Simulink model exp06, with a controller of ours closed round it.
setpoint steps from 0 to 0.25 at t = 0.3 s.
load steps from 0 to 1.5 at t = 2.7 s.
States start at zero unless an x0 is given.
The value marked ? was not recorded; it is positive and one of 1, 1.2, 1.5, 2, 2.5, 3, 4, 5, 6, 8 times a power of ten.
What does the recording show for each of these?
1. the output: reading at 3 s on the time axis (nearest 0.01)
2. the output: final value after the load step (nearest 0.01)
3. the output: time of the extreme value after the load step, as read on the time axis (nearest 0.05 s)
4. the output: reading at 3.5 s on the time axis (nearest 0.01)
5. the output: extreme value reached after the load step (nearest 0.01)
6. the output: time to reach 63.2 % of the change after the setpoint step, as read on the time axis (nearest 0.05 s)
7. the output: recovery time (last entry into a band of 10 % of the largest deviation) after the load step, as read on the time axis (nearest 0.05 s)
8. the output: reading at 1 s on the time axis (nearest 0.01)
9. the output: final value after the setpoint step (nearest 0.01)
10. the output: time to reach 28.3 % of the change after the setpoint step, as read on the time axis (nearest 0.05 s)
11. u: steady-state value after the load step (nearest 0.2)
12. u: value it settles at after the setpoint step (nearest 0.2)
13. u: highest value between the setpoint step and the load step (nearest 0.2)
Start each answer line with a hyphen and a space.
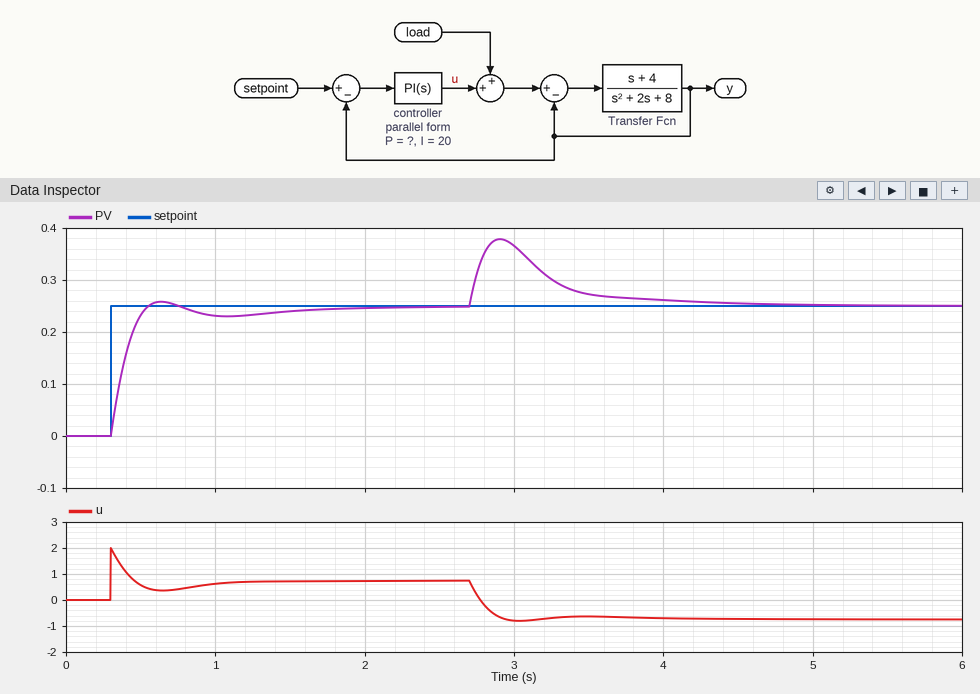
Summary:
- 0.37
- 0.25
- 2.90 s
- 0.27
- 0.38
- 0.40 s
- 3.90 s
- 0.23
- 0.25
- 0.35 s
- -0.8
- 0.8
- 2.0
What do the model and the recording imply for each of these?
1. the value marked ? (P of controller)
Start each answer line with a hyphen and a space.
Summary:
- 8
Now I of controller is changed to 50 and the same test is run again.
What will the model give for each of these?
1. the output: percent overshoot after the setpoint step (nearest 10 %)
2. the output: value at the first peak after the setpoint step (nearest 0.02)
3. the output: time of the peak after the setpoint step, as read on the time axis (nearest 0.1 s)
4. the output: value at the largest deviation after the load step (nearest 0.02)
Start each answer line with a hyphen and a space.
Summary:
- 20 %
- 0.30
- 0.6 s
- 0.36
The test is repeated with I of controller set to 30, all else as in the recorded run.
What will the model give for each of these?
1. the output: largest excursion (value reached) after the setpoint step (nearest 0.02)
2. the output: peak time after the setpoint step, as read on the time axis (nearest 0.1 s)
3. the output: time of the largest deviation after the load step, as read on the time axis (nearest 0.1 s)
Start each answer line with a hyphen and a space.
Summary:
- 0.28
- 0.6 s
- 2.9 s
